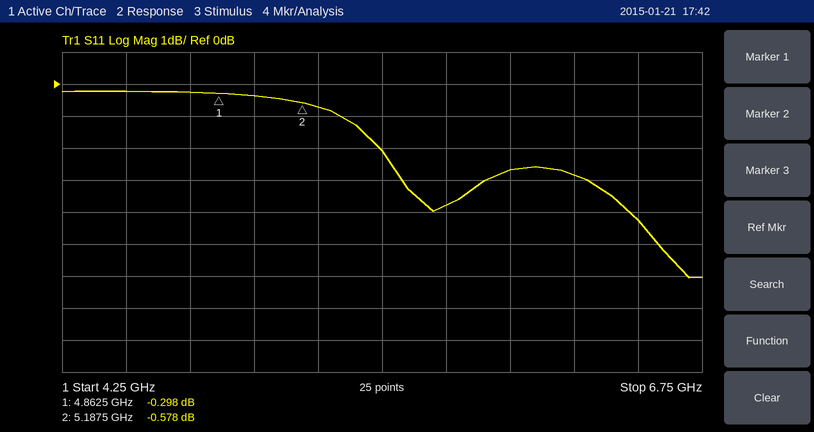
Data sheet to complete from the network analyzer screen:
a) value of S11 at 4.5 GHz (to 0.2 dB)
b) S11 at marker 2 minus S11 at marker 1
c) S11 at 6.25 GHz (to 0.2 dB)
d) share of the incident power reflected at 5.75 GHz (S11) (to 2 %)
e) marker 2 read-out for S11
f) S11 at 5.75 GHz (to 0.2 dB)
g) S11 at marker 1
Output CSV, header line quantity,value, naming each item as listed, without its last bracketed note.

quantity,value
value of S11 at 4.5 GHz,-0.2 dB
S11 at marker 2 minus S11 at marker 1,-0.280 dB
S11 at 6.25 GHz,-2.8 dB
share of the incident power reflected at 5.75 GHz (S11),42 %
marker 2 read-out for S11,-0.578 dB
S11 at 5.75 GHz,-3.8 dB
S11 at marker 1,-0.298 dB
